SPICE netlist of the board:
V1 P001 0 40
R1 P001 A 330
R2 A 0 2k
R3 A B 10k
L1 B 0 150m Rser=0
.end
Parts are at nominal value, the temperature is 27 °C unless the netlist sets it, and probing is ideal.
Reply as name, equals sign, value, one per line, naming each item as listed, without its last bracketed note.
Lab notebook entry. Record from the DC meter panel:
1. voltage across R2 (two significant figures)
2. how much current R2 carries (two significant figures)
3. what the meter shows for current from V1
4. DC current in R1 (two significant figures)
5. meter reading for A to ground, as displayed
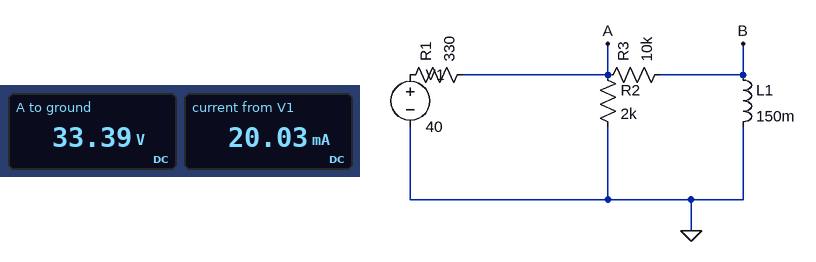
voltage across R2 = 33 V
how much current R2 carries = 17 mA
what the meter shows for current from V1 = 20.03 mA
DC current in R1 = 20 mA
meter reading for A to ground, as displayed = 33.39 V
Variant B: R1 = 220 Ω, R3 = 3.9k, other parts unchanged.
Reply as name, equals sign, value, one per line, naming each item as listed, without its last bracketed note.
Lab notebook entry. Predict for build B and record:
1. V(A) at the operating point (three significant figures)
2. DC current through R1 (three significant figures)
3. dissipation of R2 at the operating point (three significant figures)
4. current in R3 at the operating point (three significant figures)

V(A) at the operating point = 34.3 V
DC current through R1 = 25.9 mA
dissipation of R2 at the operating point = 588 mW
current in R3 at the operating point = 8.79 mA
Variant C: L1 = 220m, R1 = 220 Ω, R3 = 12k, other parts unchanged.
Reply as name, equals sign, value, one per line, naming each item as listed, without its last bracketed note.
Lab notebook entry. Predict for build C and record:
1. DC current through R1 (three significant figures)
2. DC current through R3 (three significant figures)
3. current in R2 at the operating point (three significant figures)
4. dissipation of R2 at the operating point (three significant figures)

DC current through R1 = 20.7 mA
DC current through R3 = 2.95 mA
current in R2 at the operating point = 17.7 mA
dissipation of R2 at the operating point = 628 mW
